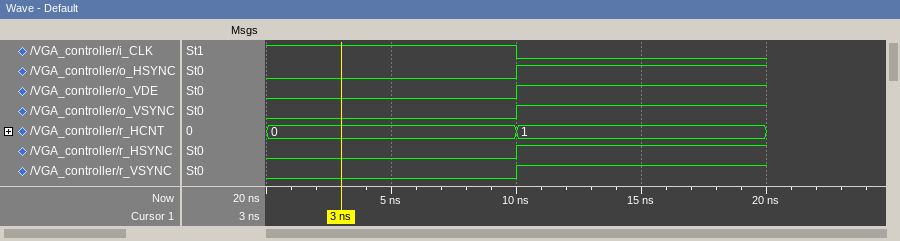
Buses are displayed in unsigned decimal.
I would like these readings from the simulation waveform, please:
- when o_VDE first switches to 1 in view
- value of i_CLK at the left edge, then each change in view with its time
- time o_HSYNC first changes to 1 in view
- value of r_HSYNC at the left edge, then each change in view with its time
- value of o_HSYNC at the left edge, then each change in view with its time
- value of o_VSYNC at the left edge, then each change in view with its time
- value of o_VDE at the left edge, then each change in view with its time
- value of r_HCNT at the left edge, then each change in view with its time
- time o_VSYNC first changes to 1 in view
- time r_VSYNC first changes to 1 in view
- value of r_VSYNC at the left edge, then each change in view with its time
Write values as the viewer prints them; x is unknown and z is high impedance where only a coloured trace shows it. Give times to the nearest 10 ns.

10 ns
1, 0 at 10 ns
10 ns
0, 1 at 10 ns
0, 1 at 10 ns
0, 1 at 10 ns
0, 1 at 10 ns
0, 1 at 10 ns
10 ns
10 ns
0, 1 at 10 ns
